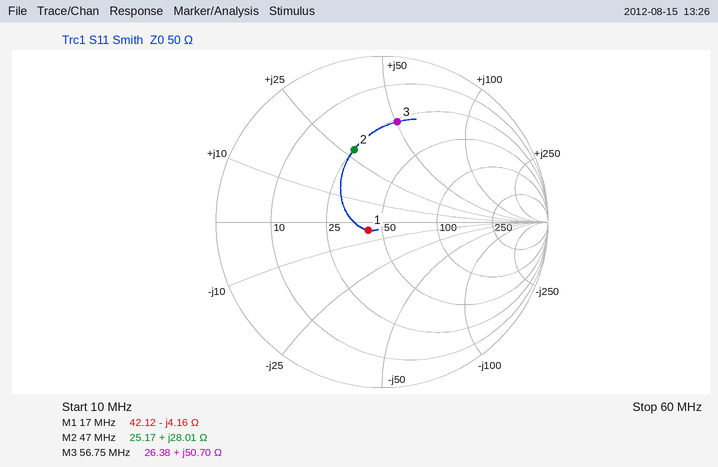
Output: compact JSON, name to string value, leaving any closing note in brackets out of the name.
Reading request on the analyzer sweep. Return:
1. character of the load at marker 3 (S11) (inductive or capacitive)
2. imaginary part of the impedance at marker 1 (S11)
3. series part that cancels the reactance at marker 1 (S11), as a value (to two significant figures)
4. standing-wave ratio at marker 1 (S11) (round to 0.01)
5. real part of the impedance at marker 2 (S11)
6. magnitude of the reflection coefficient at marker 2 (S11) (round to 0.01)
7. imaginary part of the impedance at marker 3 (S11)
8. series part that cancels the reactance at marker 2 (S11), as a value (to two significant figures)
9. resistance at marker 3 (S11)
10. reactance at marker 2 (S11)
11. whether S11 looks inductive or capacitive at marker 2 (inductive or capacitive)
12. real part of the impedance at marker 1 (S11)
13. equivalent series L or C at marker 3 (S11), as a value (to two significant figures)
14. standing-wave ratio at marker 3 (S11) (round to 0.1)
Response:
{"character of the load at marker 3 (S11)": "inductive", "imaginary part of the impedance at marker 1": "-4.16 Ω", "series part that cancels the reactance at marker 1 (S11), as a value": "39 nH", "standing-wave ratio at marker 1 (S11)": "1.21", "real part of the impedance at marker 2": "25.17 Ω", "magnitude of the reflection coefficient at marker 2 (S11)": "0.47", "imaginary part of the impedance at marker 3": "+50.70 Ω", "series part that cancels the reactance at marker 2 (S11), as a value": "120 pF", "resistance at marker 3": "26.38 Ω", "reactance at marker 2": "+28.01 Ω", "whether S11 looks inductive or capacitive at marker 2": "inductive", "real part of the impedance at marker 1": "42.12 Ω", "equivalent series L or C at marker 3 (S11), as a value": "140 nH", "standing-wave ratio at marker 3 (S11)": "4.1"}
